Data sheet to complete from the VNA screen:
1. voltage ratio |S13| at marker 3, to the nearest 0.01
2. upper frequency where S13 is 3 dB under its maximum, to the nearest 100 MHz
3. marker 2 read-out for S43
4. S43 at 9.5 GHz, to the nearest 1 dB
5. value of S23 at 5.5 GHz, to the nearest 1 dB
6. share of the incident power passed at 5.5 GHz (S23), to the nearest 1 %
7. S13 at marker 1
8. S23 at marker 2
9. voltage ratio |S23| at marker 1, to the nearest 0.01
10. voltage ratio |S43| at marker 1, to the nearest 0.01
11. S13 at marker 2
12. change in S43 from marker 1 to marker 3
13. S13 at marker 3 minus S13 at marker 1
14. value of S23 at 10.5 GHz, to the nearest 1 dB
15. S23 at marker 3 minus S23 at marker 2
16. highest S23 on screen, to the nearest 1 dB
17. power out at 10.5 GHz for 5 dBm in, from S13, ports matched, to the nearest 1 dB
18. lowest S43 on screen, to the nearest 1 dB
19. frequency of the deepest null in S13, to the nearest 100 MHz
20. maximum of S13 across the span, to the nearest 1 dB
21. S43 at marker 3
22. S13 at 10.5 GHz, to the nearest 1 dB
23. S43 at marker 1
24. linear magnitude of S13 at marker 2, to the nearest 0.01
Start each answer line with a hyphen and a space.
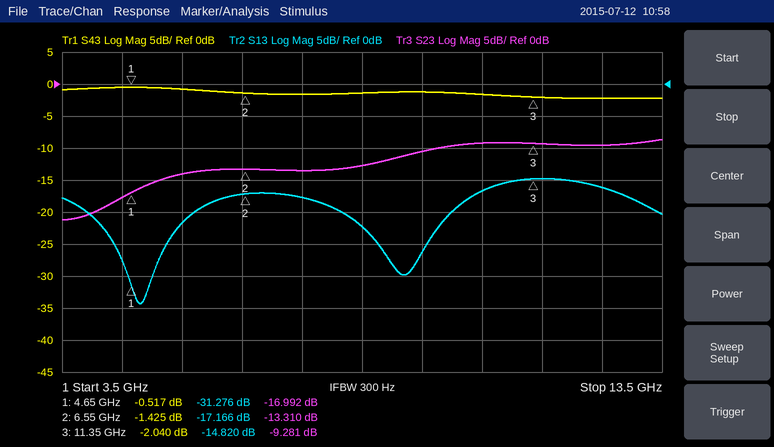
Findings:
- 0.18
- 13.0 GHz
- -1.425 dB
- -1 dB
- -14 dB
- 4 %
- -31.276 dB
- -13.310 dB
- 0.14
- 0.94
- -17.166 dB
- -1.523 dB
- 16.456 dB
- -9 dB
- 4.029 dB
- -9 dB
- -12 dBm
- -2 dB
- 4.8 GHz
- -15 dB
- -2.040 dB
- -17 dB
- -0.517 dB
- 0.14
